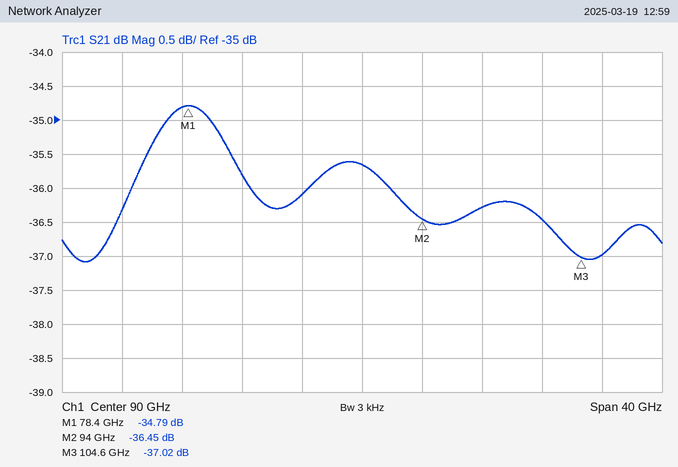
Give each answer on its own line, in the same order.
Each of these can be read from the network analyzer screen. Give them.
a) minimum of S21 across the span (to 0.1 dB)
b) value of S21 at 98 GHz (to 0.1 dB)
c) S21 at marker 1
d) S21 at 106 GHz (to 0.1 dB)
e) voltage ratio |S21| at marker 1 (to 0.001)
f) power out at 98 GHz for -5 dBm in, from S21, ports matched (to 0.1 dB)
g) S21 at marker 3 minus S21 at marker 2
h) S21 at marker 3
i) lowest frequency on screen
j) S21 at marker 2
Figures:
-37.1 dB
-36.3 dB
-34.79 dB
-37.0 dB
0.018
-41.3 dBm
-0.57 dB
-37.02 dB
70 GHz
-36.45 dB
